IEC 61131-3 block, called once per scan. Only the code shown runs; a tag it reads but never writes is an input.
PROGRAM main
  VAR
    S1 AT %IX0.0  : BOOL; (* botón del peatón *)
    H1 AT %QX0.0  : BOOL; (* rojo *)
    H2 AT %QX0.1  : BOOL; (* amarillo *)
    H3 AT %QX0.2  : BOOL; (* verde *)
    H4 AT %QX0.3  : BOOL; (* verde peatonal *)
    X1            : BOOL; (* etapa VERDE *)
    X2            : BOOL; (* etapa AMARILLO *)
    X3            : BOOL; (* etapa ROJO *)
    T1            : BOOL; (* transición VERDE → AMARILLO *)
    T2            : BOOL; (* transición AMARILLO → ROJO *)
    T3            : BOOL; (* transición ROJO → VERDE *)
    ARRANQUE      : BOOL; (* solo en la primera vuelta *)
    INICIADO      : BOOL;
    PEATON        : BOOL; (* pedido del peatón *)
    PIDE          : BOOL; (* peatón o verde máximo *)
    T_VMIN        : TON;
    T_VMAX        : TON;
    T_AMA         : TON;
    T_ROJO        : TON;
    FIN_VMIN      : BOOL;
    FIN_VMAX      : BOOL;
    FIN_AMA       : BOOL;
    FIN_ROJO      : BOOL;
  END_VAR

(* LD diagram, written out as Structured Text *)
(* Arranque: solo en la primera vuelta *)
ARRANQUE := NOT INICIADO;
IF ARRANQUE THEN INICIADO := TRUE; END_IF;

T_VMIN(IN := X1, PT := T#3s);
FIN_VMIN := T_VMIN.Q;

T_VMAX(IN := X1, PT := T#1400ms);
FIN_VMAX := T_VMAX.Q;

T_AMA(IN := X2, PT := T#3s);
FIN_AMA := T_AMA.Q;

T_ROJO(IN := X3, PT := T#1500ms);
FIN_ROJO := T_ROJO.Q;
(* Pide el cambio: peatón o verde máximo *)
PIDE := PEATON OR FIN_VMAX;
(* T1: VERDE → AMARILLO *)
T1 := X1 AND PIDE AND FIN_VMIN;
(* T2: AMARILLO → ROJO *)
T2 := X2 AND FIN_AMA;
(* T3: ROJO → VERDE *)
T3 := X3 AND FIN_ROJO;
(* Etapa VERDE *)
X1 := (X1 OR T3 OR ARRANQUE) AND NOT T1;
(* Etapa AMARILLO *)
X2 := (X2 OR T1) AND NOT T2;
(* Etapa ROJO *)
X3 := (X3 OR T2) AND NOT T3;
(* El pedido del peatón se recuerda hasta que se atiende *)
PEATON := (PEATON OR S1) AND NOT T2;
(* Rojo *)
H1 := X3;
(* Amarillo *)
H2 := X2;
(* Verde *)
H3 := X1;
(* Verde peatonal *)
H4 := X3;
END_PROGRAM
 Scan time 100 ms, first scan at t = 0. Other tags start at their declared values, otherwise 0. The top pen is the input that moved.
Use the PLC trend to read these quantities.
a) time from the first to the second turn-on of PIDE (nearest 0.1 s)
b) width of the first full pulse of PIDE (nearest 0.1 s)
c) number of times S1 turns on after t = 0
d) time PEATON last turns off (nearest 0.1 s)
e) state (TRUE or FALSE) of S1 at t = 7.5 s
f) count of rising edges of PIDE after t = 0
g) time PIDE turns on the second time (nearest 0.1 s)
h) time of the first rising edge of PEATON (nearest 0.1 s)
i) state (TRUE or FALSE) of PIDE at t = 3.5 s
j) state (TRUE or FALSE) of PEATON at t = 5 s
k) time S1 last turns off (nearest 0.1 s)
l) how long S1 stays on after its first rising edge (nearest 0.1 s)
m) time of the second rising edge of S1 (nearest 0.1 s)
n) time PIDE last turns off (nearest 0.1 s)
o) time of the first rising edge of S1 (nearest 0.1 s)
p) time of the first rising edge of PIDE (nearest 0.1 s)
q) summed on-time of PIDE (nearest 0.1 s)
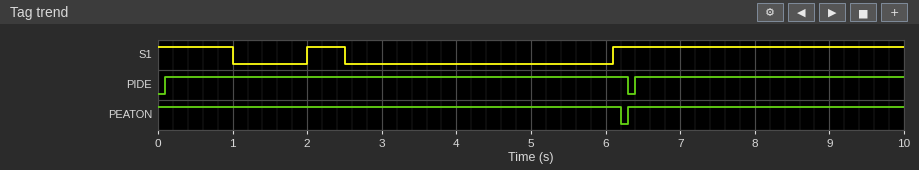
6.3 s
6.2 s
2
6.2 s
TRUE
2
6.4 s
6.3 s
TRUE
TRUE
2.5 s
0.5 s
6.1 s
6.3 s
2.0 s
0.1 s
9.8 s
